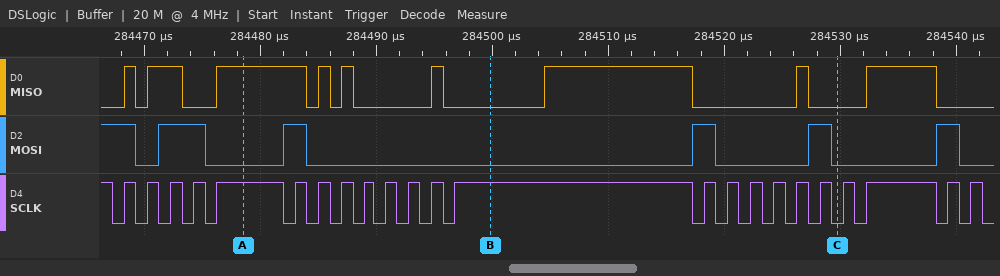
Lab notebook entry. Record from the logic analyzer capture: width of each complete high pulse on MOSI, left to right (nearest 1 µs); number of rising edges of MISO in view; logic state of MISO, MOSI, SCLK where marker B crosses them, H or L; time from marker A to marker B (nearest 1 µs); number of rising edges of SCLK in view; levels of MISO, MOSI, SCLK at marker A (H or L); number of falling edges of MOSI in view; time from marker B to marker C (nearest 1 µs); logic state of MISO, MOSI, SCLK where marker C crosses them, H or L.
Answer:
4 µs, 2 µs, 2 µs, 2 µs, 2 µs
9
MISO=L, MOSI=L, SCLK=H
21 µs
23
MISO=H, MOSI=L, SCLK=H
6
30 µs
MISO=L, MOSI=L, SCLK=L
